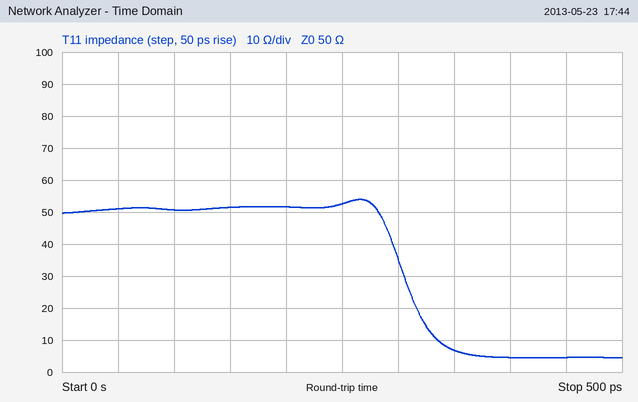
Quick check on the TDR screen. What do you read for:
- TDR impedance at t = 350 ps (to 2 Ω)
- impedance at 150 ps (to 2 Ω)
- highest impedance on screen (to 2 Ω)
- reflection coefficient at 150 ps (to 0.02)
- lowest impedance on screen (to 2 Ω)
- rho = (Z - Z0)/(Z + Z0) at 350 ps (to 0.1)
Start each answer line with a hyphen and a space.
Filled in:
- 6 Ω
- 52 Ω
- 54 Ω
- +0.02
- 4 Ω
- -0.8
